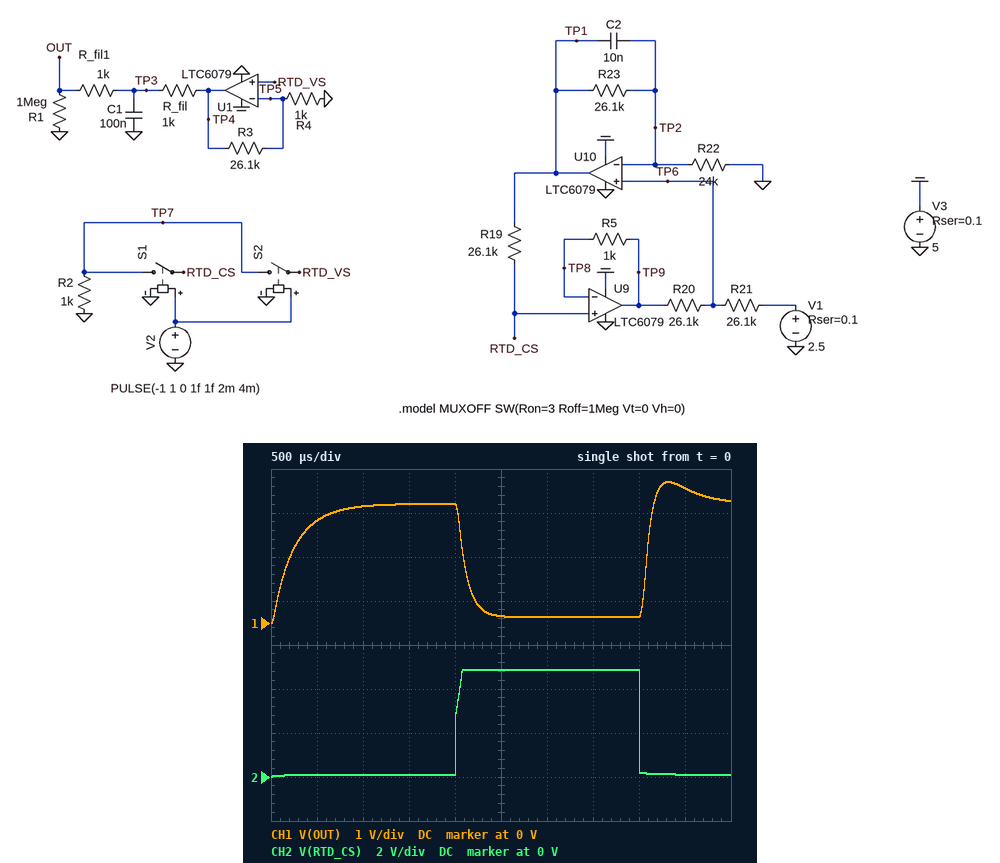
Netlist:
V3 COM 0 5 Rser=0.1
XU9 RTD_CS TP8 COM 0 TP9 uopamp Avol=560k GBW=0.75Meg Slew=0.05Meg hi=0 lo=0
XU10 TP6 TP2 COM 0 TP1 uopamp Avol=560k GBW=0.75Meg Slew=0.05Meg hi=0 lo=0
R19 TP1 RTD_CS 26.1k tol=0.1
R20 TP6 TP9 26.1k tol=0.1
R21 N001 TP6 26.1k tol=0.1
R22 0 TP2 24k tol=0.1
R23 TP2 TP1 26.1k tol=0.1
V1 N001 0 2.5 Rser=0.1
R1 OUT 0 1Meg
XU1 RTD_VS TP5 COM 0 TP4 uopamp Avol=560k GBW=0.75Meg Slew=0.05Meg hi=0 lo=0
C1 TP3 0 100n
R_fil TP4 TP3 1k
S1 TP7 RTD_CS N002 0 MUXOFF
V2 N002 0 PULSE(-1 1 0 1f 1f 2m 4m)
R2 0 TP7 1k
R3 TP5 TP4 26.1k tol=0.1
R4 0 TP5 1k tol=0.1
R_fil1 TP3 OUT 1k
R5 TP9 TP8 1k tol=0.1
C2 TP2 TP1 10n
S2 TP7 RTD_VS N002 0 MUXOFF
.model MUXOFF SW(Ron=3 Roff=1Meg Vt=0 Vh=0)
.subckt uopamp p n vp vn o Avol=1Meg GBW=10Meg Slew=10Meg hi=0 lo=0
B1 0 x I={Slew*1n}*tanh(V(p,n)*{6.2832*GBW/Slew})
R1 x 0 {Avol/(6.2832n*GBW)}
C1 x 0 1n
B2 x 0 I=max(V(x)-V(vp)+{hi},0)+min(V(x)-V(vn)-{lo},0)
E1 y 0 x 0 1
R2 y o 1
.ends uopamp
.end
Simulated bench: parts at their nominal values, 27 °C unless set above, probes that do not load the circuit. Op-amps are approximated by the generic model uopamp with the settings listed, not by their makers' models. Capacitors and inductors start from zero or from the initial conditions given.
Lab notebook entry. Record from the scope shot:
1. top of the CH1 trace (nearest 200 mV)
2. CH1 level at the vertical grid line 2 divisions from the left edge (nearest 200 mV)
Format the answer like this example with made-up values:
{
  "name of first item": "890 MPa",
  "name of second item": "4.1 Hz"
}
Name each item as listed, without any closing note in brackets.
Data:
{
  "top of the CH1 trace": "3.2 V",
  "CH1 level at the vertical grid line 2 divisions from the left edge": "2.6 V"
}
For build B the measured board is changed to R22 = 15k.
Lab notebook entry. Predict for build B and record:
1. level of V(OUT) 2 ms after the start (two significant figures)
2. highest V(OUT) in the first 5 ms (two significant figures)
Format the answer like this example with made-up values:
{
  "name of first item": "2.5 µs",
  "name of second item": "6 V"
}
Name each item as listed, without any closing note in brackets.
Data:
{
  "level of V(OUT) 2 ms after the start": "3.6 V",
  "highest V(OUT) in the first 5 ms": "3.9 V"
}
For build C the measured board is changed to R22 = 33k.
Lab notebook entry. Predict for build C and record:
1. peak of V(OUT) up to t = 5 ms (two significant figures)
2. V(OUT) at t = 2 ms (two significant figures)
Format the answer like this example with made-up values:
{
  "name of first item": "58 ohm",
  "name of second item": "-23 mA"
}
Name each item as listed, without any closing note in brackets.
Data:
{
  "peak of V(OUT) up to t = 5 ms": "2.8 V",
  "V(OUT) at t = 2 ms": "2.3 V"
}
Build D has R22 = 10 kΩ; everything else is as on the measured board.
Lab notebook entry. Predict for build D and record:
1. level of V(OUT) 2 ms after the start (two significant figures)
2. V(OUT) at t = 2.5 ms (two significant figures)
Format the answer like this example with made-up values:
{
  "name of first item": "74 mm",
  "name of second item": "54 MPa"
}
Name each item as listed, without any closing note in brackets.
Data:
{
  "level of V(OUT) 2 ms after the start": "4.8 V",
  "V(OUT) at t = 2.5 ms": "180 mV"
}
